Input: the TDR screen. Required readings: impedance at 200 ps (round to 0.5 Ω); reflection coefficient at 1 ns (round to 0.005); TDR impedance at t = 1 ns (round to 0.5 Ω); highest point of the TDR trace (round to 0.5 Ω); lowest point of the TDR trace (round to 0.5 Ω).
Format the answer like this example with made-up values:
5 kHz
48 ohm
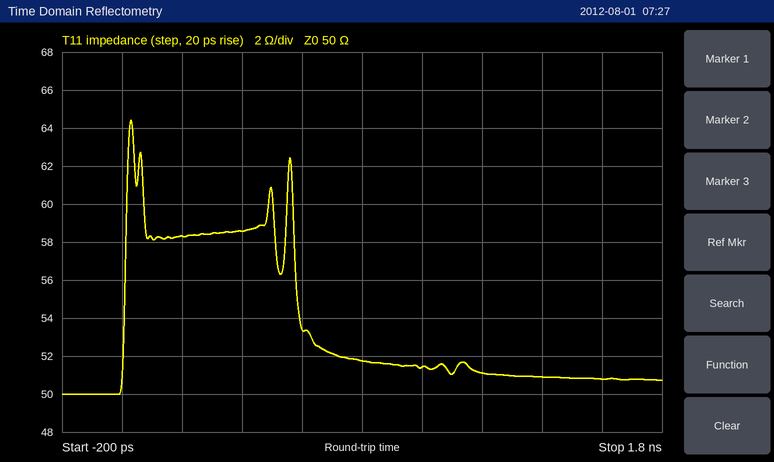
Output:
58.5 Ω
+0.015
51.5 Ω
64.5 Ω
50.0 Ω
